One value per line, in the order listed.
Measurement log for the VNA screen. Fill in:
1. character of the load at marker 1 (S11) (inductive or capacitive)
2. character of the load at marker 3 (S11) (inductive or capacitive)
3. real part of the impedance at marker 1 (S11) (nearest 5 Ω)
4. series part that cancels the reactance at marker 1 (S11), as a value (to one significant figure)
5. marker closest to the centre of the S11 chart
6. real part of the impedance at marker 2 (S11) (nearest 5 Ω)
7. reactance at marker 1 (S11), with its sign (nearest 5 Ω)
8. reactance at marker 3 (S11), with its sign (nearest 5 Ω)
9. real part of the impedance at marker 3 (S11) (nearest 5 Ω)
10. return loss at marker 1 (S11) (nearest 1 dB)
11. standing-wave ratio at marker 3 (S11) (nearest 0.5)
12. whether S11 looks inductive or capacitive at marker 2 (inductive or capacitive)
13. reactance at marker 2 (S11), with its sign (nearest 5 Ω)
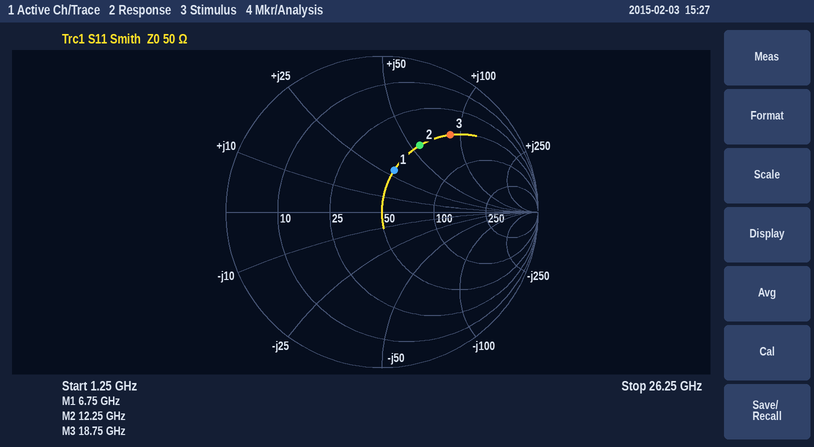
inductive
inductive
50 Ω
800 fF
marker 1
50 Ω
+30 Ω
+90 Ω
50 Ω
11 dB
5.0
inductive
+55 Ω
